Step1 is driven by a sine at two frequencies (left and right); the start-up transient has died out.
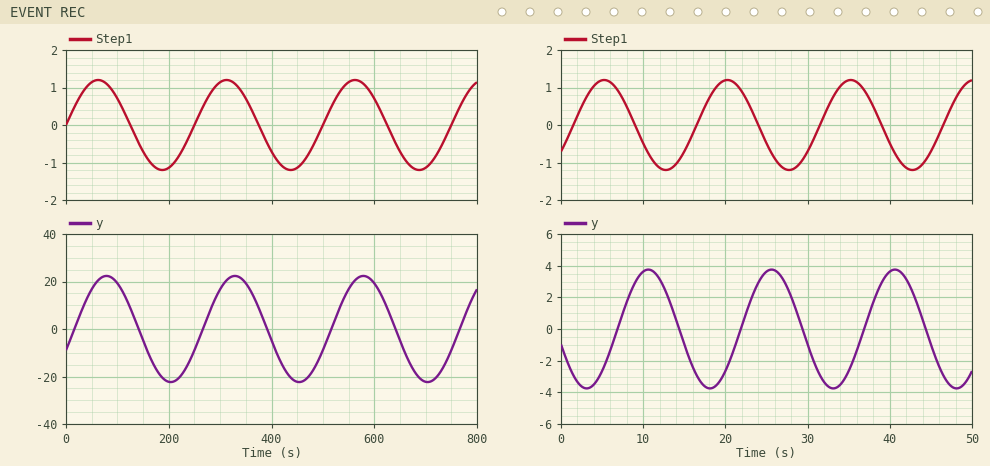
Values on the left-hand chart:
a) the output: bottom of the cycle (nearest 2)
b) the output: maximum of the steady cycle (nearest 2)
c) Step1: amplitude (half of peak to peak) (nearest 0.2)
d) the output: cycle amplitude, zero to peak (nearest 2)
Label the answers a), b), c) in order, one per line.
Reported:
a) -22
b) 22
c) 1.2
d) 22
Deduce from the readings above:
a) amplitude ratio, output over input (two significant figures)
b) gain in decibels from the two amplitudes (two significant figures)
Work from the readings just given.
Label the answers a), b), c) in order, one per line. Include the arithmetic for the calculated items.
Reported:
a) 22 / 1.2 = 18
b) 20 log10(22 / 1.2) = 25 dB
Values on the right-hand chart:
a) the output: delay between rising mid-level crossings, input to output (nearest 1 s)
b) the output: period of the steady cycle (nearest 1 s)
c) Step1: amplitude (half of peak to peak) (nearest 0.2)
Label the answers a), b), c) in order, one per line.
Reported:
a) 5 s
b) 15 s
c) 1.2
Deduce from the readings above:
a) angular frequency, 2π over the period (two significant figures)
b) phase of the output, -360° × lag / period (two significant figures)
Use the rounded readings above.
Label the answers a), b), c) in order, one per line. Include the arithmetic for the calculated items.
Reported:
a) 2π / 15 = 0.42 rad/s
b) -360 × 5 / 15 = -120°
